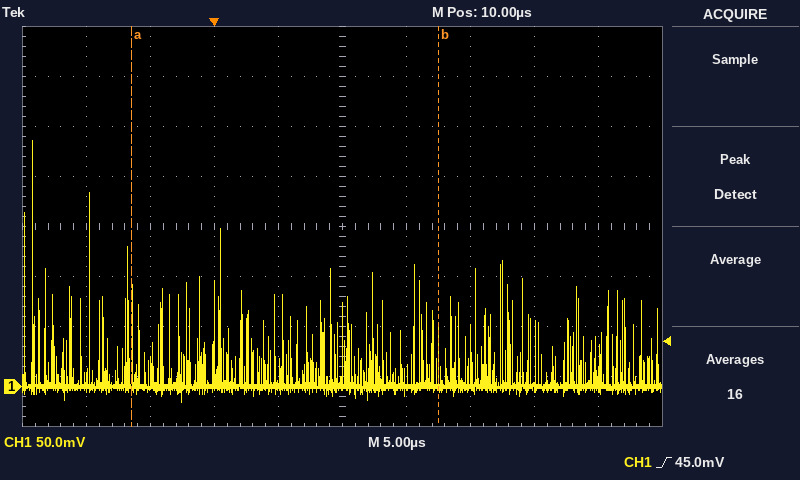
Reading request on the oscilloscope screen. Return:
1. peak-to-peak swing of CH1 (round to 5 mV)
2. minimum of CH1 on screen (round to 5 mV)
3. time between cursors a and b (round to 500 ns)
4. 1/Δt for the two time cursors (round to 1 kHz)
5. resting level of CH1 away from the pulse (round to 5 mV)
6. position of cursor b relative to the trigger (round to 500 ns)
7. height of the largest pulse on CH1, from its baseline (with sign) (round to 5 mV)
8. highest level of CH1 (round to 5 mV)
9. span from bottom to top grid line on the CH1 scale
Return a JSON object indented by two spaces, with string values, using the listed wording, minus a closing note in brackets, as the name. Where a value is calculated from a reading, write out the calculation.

{
  "peak-to-peak swing of CH1": "245 mV − (-15 mV) = 260 mV",
  "minimum of CH1 on screen": "-15 mV",
  "time between cursors a and b": "24.0 µs",
  "1/Δt for the two time cursors": "1 / 24.0 µs ≈ 42 kHz",
  "resting level of CH1 away from the pulse": "0 mV",
  "position of cursor b relative to the trigger": "+17.5 µs",
  "height of the largest pulse on CH1, from its baseline (with sign)": "245 mV − (0 mV) = +245 mV",
  "highest level of CH1": "245 mV",
  "span from bottom to top grid line on the CH1 scale": "400 mV"
}
